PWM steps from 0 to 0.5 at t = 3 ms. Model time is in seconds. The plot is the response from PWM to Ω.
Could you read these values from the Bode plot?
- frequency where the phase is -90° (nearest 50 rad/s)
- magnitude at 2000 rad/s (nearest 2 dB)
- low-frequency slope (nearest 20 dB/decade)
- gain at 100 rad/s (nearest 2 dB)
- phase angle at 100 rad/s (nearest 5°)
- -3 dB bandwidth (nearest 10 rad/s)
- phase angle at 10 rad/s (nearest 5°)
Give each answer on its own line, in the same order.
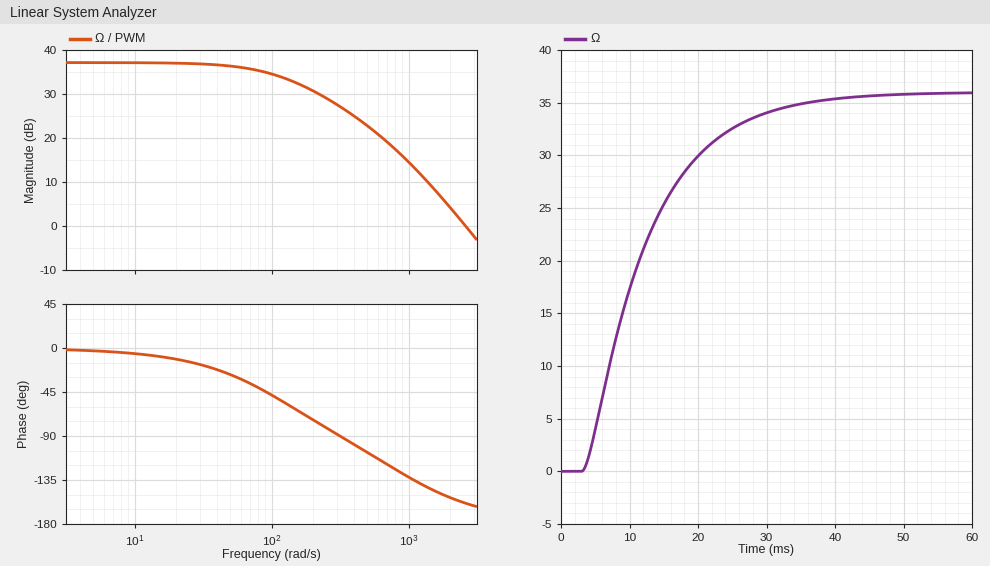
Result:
300 rad/s
4 dB
0 dB/decade
34 dB
-50°
110 rad/s
-5°
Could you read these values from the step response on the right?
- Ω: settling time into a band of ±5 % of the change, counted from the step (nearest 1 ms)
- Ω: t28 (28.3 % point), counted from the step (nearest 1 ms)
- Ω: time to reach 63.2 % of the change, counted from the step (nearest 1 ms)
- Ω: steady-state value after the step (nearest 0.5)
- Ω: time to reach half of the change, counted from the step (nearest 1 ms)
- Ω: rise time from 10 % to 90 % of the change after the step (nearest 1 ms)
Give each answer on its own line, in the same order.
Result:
28 ms
4 ms
10 ms
36.0
7 ms
20 ms
